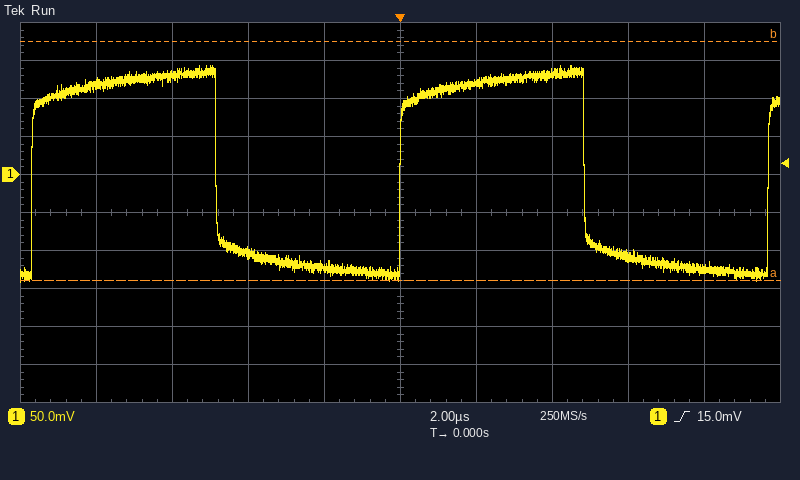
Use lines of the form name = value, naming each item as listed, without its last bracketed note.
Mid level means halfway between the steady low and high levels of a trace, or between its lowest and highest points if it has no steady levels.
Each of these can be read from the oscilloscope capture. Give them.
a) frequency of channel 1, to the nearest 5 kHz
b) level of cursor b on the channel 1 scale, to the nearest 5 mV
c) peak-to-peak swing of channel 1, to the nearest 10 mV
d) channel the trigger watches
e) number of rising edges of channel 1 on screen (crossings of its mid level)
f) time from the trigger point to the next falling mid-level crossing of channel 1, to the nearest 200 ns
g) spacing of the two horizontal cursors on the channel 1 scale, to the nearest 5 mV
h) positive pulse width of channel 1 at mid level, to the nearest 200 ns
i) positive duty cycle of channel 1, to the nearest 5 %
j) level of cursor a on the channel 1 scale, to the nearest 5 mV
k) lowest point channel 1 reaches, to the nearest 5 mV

frequency of channel 1, to the nearest 5 kHz = 105 kHz
level of cursor b on the channel 1 scale, to the nearest 5 mV = 175 mV
peak-to-peak swing of channel 1, to the nearest 10 mV = 280 mV
channel the trigger watches = channel 1
number of rising edges of channel 1 on screen = 3
time from the trigger point to the next falling mid-level crossing of channel 1, to the nearest 200 ns = 4.8 µs
spacing of the two horizontal cursors on the channel 1 scale, to the nearest 5 mV = 315 mV
positive pulse width of channel 1 at mid level, to the nearest 200 ns = 4.8 µs
positive duty cycle of channel 1, to the nearest 5 % = 50 %
level of cursor a on the channel 1 scale, to the nearest 5 mV = -140 mV
lowest point channel 1 reaches, to the nearest 5 mV = -140 mV
